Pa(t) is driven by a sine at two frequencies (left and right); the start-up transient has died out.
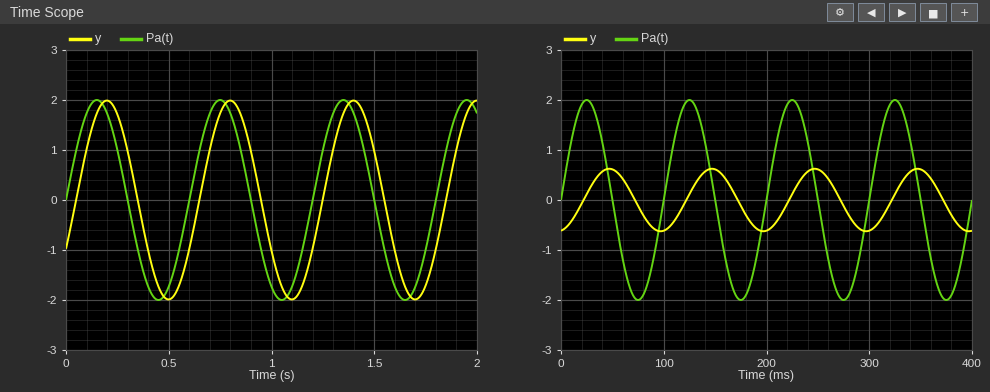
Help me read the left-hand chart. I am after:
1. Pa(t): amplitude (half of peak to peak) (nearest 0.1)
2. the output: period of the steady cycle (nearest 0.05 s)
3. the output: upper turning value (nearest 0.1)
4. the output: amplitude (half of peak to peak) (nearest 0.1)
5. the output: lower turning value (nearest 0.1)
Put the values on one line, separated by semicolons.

2.0; 0.60 s; 2.0; 2.0; -2.0
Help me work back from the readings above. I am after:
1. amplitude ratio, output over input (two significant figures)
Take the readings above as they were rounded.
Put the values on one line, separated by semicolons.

1.0
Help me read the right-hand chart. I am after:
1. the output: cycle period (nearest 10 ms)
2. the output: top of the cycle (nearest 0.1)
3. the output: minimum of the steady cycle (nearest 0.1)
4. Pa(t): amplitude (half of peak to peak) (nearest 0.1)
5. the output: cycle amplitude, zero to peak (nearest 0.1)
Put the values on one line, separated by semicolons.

100 ms; 0.6; -0.6; 2.0; 0.6
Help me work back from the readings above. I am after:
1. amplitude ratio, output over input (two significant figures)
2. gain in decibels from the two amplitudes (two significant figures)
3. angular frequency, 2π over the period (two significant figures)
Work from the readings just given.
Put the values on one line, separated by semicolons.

0.30; -10 dB; 0.063 rad/ms
